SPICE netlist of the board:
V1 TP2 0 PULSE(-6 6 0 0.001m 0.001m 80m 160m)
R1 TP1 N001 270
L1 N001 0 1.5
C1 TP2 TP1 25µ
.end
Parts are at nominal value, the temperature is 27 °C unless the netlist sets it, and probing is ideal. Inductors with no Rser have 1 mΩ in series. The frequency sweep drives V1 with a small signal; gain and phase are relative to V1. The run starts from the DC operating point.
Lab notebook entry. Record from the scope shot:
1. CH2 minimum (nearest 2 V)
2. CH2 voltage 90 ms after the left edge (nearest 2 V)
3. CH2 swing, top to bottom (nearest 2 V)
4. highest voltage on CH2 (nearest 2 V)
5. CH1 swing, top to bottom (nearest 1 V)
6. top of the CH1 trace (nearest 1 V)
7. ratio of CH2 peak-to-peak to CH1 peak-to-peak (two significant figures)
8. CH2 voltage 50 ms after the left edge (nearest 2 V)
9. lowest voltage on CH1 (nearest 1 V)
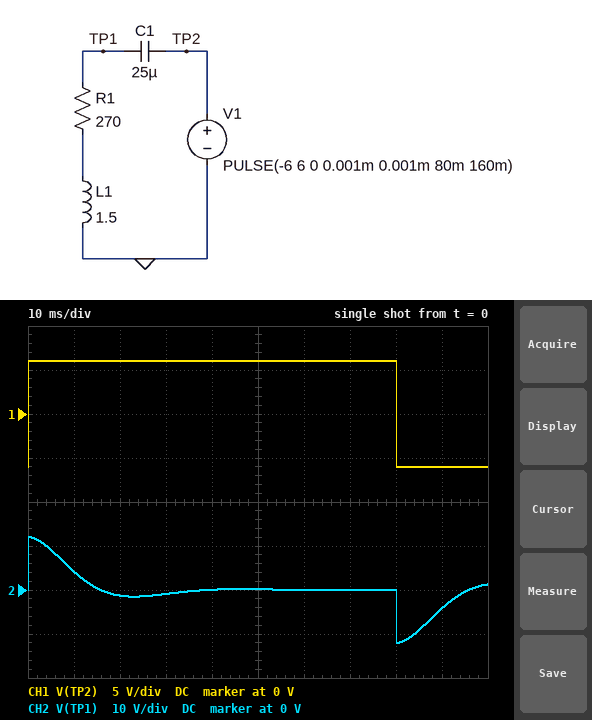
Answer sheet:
-12 V
-4 V
24 V
12 V
12 V
6 V
2.0
0 V
-6 V
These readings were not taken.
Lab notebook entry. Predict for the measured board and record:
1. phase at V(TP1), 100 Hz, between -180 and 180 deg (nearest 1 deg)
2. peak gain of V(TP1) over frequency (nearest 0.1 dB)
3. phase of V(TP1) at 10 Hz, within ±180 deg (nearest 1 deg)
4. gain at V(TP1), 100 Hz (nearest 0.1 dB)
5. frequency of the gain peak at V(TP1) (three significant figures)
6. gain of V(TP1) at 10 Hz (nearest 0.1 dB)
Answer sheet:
1 deg
2.9 dB
83 deg
0.6 dB
31.0 Hz
-6.5 dB
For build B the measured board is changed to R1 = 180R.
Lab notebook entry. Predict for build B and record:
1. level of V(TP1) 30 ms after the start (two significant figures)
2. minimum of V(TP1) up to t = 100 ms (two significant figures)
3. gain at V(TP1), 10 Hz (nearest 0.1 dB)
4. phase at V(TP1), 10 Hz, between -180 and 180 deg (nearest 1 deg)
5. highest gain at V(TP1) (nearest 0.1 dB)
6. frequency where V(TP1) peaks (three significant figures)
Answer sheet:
-1.1 V
-12 V
-9.0 dB
99 deg
4.8 dB
28.7 Hz
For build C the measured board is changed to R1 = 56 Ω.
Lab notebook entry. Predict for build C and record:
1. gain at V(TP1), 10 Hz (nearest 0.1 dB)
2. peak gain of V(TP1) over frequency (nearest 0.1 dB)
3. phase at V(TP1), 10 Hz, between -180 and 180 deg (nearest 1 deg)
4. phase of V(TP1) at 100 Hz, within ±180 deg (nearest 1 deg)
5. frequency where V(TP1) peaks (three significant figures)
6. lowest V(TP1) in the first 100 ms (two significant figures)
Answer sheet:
-13.9 dB
13.1 dB
143 deg
0 deg
26.3 Hz
-9.5 V
